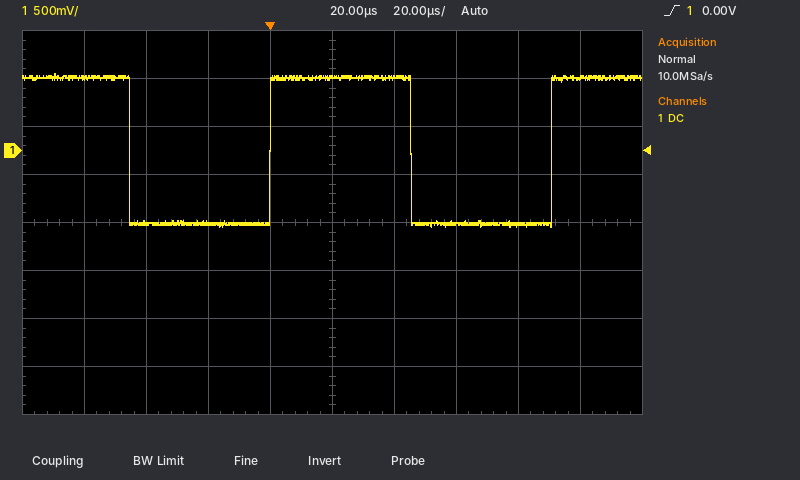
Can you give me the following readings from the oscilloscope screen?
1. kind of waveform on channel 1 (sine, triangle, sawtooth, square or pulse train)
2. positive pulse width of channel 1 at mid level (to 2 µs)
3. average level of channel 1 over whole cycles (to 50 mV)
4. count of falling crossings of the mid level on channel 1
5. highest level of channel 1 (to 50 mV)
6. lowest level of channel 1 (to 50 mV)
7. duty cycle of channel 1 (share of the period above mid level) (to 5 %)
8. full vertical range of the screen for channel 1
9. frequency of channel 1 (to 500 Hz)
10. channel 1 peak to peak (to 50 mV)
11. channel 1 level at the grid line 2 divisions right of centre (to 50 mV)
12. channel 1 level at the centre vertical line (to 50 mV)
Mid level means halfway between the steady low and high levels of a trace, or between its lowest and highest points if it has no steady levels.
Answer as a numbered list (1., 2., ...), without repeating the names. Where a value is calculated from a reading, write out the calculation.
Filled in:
1. square
2. 46 µs
3. -800 mV + 0.5 × (800 mV − (-800 mV)) ≈ 0 mV
4. 2
5. 800 mV
6. -800 mV
7. 50 %
8. 4 V
9. 11.0 kHz
10. 800 mV − (-800 mV) = 1.60 V
11. -750 mV
12. 750 mV
